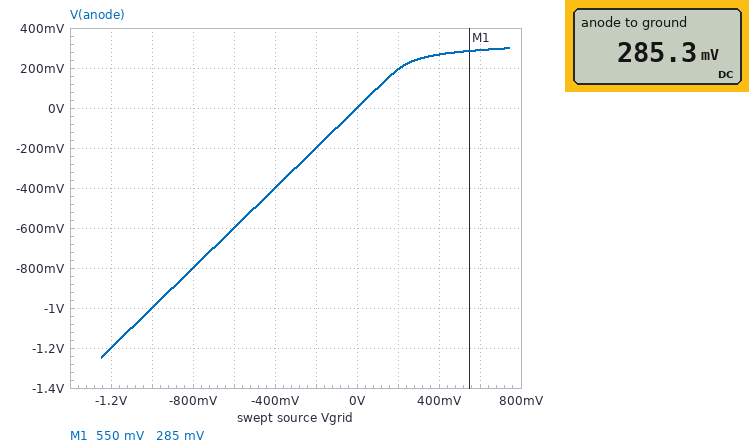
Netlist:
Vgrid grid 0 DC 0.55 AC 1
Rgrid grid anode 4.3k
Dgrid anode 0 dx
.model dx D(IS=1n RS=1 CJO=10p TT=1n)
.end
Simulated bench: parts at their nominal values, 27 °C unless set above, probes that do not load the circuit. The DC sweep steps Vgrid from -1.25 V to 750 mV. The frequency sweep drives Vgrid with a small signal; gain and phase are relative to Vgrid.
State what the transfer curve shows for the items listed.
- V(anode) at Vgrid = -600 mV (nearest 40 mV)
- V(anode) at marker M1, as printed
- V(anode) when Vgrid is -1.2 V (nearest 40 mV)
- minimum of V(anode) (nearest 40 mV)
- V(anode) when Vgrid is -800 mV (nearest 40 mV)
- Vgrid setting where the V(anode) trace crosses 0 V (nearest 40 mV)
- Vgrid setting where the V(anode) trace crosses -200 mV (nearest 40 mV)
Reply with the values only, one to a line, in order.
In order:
-600 mV
285 mV
-1.20 V
-1.24 V
-800 mV
0 V
-200 mV
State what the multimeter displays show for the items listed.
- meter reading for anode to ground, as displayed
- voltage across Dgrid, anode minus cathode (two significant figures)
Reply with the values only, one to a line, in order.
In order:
285.3 mV
290 mV
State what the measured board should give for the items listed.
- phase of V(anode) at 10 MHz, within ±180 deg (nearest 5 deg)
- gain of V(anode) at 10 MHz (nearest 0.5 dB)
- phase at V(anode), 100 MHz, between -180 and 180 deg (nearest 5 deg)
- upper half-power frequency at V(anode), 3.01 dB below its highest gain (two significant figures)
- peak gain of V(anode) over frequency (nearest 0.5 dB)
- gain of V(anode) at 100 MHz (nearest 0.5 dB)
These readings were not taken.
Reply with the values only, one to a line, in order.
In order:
-20 deg
-21.5 dB
-75 deg
29 MHz
-21.0 dB
-32.0 dB
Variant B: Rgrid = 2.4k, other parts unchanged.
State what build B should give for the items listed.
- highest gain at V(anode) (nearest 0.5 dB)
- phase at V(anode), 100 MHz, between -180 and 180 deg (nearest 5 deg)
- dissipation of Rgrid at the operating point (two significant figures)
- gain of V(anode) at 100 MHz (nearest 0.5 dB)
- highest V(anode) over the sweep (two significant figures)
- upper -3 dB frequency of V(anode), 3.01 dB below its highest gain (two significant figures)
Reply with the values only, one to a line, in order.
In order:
-20.5 dB
-65 deg
26 µW
-28.5 dB
310 mV
44 MHz
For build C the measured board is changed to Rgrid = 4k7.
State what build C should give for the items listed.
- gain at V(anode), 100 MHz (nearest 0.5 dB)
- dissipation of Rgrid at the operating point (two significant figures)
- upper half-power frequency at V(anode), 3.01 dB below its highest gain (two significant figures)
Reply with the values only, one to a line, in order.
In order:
-32.5 dB
15 µW
27 MHz
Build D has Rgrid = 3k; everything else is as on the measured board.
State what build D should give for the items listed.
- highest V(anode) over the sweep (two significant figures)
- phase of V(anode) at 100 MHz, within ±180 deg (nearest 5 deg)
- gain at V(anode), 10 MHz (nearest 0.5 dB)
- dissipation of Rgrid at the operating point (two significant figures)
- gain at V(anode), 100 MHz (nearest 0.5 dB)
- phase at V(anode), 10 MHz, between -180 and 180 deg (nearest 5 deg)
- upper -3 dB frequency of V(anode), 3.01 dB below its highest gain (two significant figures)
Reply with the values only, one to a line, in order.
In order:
310 mV
-70 deg
-21.0 dB
22 µW
-29.5 dB
-15 deg
38 MHz
